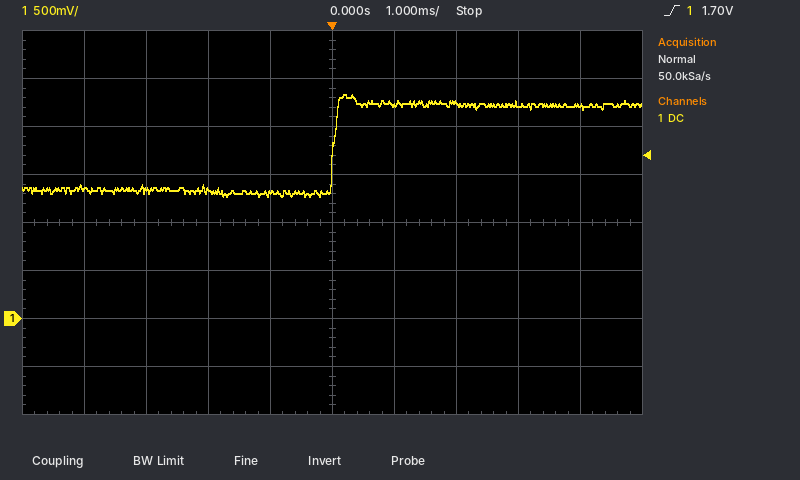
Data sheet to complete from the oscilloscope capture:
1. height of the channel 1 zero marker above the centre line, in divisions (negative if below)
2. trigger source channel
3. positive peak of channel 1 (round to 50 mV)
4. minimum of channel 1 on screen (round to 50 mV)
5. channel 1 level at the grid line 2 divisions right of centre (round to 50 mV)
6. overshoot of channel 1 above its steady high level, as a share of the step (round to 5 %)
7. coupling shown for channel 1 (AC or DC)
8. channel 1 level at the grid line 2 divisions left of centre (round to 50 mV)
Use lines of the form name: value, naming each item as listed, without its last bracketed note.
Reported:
height of the channel 1 zero marker above the centre line, in divisions: -2.0 div
trigger source channel: channel 1
positive peak of channel 1: 2.35 V
minimum of channel 1 on screen: 1.25 V
channel 1 level at the grid line 2 divisions right of centre: 2.25 V
overshoot of channel 1 above its steady high level, as a share of the step: 10 %
coupling shown for channel 1: DC
channel 1 level at the grid line 2 divisions left of centre: 1.35 V
